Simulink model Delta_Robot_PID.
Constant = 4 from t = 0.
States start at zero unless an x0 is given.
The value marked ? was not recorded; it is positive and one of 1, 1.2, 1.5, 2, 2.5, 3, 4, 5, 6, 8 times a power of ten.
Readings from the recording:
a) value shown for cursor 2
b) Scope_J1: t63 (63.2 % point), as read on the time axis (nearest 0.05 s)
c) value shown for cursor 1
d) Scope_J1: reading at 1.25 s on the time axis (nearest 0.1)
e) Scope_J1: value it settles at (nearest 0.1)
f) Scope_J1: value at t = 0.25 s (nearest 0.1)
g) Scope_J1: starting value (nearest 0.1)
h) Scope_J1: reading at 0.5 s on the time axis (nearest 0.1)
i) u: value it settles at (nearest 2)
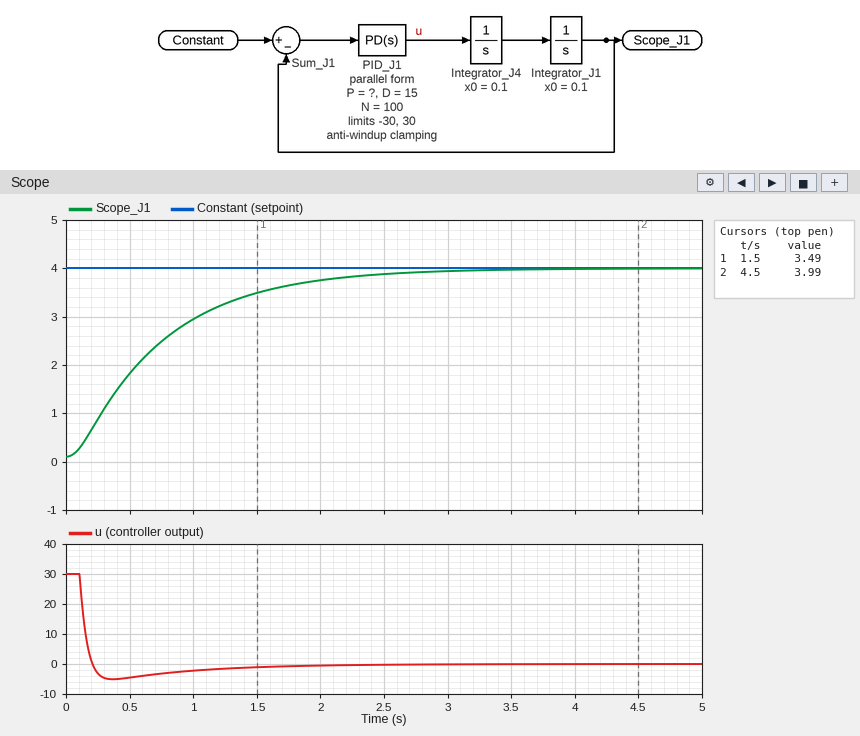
3.99
0.80 s
3.49
3.3
4.0
0.9
0.1
1.8
0
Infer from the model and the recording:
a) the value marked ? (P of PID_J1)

20
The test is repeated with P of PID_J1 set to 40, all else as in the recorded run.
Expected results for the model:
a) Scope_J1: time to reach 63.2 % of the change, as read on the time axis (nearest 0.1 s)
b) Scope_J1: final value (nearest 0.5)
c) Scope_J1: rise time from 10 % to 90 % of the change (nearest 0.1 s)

0.5 s
4.0
0.7 s
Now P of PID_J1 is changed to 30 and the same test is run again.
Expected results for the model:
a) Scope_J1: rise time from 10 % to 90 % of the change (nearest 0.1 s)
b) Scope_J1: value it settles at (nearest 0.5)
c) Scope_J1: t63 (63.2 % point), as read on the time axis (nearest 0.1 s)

1.0 s
4.0
0.6 s
